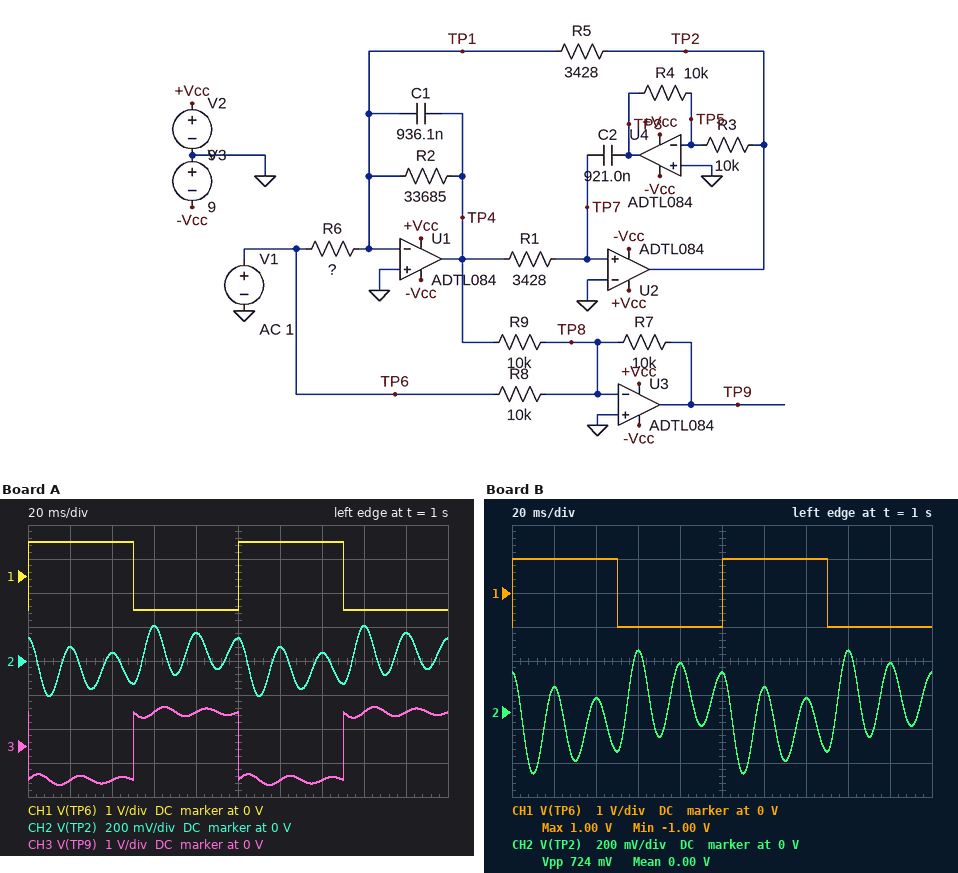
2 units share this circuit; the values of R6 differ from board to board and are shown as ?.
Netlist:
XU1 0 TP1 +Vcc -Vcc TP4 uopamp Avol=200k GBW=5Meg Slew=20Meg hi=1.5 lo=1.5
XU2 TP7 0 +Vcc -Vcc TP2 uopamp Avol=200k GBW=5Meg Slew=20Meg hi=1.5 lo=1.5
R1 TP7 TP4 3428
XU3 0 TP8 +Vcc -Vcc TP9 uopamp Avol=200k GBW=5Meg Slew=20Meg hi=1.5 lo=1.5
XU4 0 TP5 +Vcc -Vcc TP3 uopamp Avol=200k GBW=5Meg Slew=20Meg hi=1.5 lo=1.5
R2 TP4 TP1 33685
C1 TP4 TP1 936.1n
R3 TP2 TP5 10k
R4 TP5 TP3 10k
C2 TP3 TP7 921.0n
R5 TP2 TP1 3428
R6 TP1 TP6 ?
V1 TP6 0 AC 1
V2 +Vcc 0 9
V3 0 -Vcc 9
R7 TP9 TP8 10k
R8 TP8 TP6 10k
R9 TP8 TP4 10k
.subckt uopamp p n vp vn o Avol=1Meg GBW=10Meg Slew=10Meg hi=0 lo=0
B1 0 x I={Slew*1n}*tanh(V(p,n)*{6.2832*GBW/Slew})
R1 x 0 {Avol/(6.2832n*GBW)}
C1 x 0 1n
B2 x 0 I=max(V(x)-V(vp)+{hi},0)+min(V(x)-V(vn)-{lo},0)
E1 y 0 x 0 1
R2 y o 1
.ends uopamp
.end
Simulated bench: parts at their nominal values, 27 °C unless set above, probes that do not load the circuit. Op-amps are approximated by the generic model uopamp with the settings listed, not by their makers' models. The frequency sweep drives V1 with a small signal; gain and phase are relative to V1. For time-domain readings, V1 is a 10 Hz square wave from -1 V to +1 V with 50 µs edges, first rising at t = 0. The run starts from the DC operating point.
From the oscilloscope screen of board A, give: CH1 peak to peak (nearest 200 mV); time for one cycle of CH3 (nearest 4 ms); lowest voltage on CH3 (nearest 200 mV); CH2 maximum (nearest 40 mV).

2.0 V
100 ms
-1.2 V
200 mV
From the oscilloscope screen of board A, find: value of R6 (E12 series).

68 kΩ
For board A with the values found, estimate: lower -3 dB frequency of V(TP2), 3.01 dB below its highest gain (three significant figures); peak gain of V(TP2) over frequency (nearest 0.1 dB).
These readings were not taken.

47.3 Hz
-6.0 dB
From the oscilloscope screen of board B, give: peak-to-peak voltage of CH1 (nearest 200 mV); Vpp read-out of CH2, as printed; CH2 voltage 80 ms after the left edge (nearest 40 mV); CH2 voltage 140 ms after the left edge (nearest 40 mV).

2.0 V
724 mV
280 mV
80 mV
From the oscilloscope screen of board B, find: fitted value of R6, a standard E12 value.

39 kΩ
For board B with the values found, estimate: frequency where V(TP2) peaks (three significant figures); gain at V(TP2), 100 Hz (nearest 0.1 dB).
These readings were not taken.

49.9 Hz
-30.7 dB
